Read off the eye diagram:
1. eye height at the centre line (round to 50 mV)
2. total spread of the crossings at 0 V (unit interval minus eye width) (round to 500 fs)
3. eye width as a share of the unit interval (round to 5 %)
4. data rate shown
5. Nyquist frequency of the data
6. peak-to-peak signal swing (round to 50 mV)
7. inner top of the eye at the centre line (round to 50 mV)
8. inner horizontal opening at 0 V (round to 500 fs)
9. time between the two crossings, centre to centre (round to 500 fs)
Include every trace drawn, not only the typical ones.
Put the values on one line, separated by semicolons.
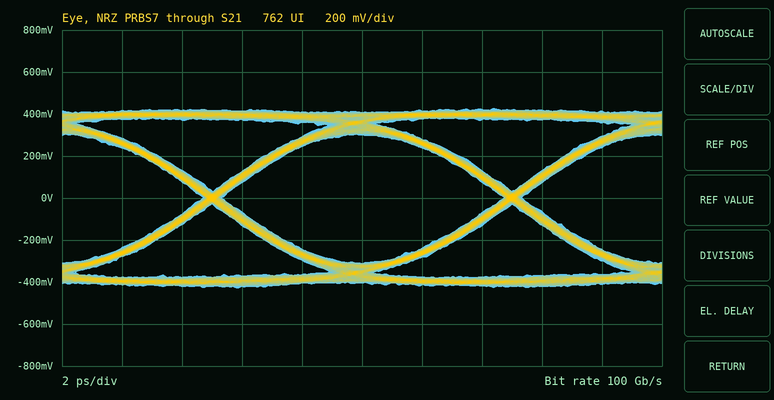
600 mV; 500 fs; 95 %; 100 Gb/s; 50 GHz; 850 mV; 300 mV; 9.5 ps; 10.0 ps
